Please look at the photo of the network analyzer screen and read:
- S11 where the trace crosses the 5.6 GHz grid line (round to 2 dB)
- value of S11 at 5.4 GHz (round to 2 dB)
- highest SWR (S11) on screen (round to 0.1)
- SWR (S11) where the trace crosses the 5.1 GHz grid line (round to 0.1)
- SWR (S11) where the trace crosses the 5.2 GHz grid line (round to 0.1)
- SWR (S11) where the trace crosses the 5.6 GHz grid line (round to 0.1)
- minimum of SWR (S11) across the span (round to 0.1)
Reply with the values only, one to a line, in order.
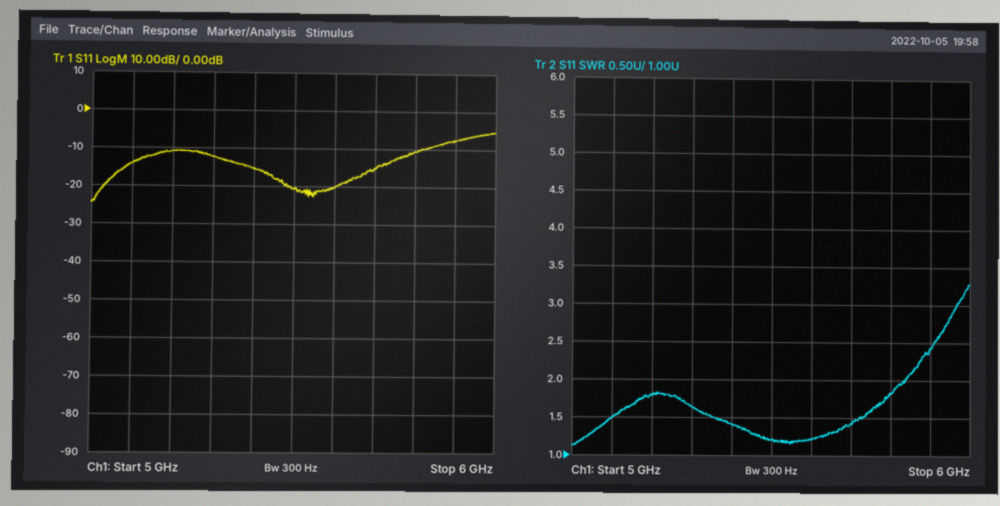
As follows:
-20 dB
-16 dB
3.3
1.5
1.8
1.2
1.1
